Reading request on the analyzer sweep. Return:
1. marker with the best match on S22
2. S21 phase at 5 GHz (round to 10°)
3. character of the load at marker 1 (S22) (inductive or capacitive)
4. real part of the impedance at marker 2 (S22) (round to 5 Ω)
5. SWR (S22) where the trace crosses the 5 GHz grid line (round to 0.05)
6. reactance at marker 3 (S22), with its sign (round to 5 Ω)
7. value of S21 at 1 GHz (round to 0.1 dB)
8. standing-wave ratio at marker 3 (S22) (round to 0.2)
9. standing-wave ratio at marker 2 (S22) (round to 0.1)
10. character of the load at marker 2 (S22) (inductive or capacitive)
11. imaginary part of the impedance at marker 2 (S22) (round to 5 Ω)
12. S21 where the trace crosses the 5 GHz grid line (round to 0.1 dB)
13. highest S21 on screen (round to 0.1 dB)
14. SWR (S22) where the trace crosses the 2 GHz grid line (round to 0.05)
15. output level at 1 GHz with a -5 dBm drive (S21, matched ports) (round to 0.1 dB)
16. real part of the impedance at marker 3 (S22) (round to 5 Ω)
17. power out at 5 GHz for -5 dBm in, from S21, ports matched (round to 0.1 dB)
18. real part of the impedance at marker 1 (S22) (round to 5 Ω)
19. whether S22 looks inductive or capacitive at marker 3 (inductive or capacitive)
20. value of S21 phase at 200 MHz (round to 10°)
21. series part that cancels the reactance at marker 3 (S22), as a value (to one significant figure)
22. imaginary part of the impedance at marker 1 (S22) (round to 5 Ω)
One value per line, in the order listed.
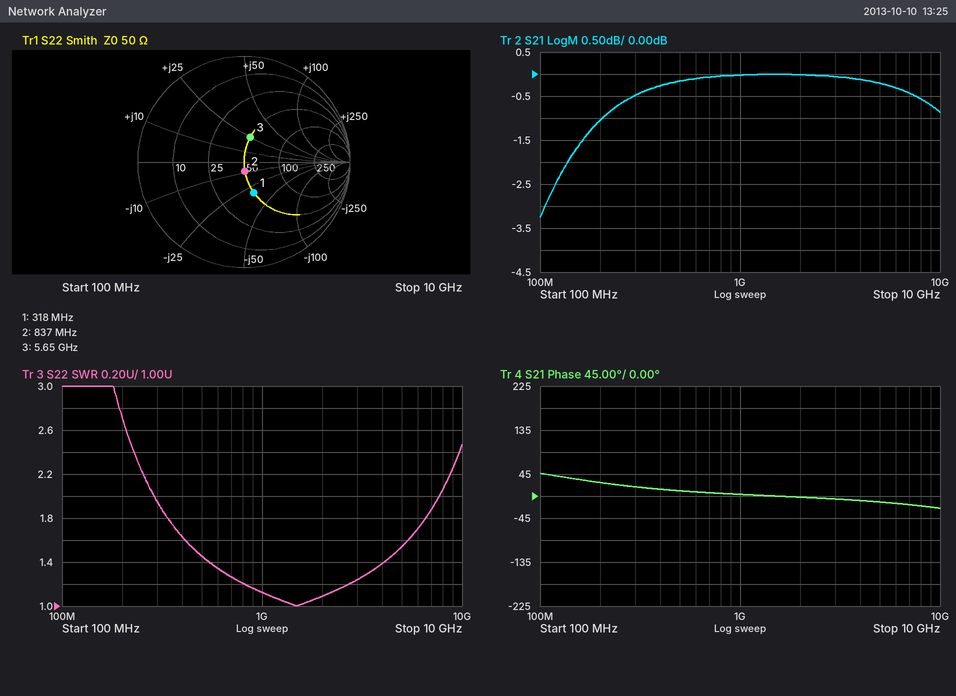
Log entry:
marker 2
-10°
capacitive
50 Ω
1.55
+25 Ω
0.0 dB
1.6
1.2
capacitive
-10 Ω
-0.2 dB
0.0 dB
1.10
-5.0 dBm
50 Ω
-5.2 dBm
50 Ω
inductive
30°
1 pF
-30 Ω
